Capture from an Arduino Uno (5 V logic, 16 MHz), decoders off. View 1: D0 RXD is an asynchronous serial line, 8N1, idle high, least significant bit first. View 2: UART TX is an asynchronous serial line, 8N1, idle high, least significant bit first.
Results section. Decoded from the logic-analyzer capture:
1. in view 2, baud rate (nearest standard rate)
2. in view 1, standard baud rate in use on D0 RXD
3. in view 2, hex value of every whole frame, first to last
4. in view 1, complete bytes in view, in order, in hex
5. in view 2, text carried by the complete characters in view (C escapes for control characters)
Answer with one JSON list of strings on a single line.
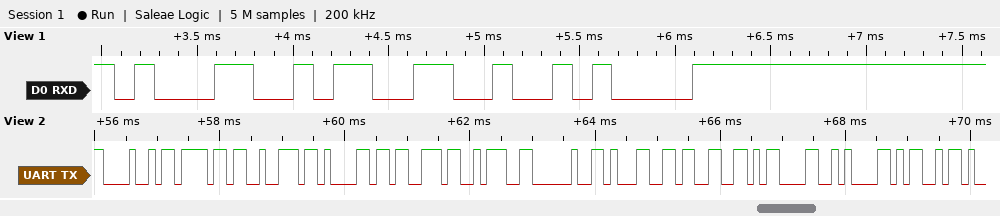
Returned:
["9600 baud", "9600 baud", "48 6F 72 61 73 3A 20 31 33 0D 0A 4D", "31 33 0A", "\"Horas: 13\\r\\nM\""]
